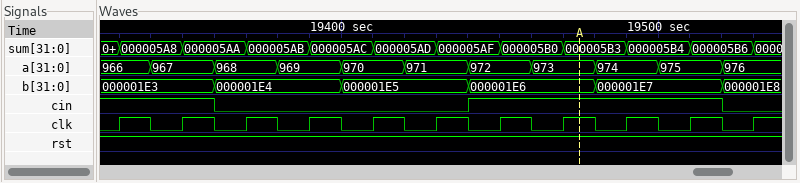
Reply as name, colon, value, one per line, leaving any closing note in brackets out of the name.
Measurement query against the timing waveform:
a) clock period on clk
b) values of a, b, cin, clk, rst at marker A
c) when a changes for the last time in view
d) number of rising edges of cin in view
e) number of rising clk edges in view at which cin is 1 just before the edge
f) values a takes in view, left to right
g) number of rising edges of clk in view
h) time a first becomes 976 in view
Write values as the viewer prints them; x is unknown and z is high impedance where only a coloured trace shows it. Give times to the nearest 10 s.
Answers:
clock period on clk: 20 s
values of a, b, cin, clk, rst at marker A: a=973, b=000001E6, cin=1, clk=1, rst=1
when a changes for the last time in view: 19520 s
number of rising edges of cin in view: 1
number of rising clk edges in view at which cin is 1 just before the edge: 6
values a takes in view, left to right: 966, 967, 968, 969, 970, 971, 972, 973, 974, 975, 976
number of rising edges of clk in view: 11
time a first becomes 976 in view: 19520 s
